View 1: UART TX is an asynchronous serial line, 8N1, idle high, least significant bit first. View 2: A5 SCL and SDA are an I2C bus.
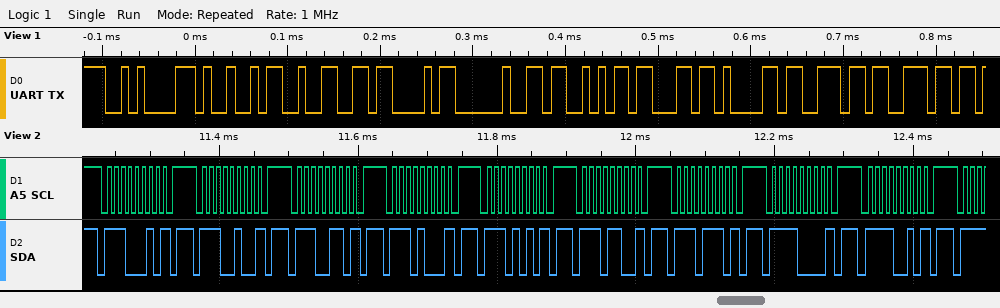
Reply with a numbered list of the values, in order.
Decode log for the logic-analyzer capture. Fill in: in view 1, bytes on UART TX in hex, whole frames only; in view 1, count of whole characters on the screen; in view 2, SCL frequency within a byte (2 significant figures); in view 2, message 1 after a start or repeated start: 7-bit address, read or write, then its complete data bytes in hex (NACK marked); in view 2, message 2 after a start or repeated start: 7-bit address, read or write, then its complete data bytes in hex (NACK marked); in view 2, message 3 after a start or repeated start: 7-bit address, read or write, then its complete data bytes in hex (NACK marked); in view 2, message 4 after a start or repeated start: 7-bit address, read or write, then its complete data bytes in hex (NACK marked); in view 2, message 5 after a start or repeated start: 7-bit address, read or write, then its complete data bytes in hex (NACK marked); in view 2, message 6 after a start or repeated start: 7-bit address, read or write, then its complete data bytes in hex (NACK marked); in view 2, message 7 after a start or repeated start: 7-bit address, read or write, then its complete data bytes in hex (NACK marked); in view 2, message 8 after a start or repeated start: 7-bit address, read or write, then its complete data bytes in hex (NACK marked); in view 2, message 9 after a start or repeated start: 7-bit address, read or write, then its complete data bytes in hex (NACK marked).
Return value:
1. 0A 49 32 43 20 53 63 61 6E 6E
2. 10
3. 100 kHz
4. 0x71 write NACK
5. 0x72 write NACK
6. 0x73 write NACK
7. 0x74 write NACK
8. 0x75 write NACK
9. 0x76 write NACK
10. 0x77 write NACK
11. 0x78 write NACK
12. 0x79 write NACK
